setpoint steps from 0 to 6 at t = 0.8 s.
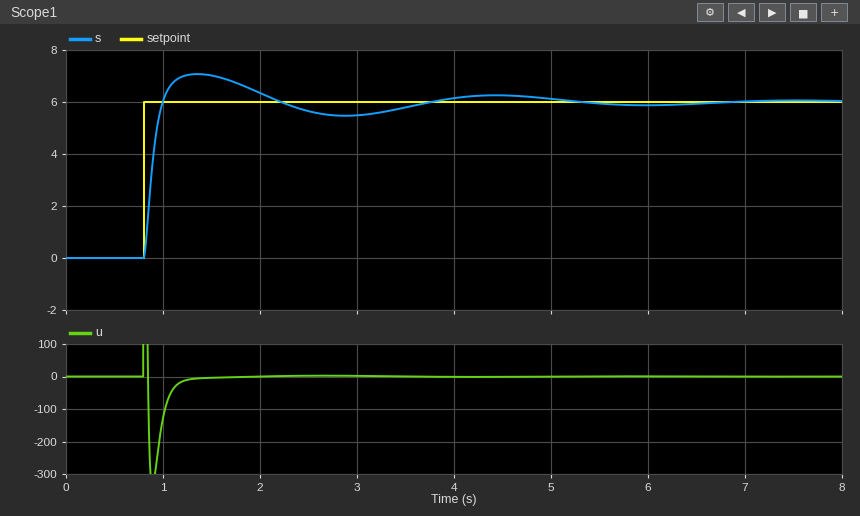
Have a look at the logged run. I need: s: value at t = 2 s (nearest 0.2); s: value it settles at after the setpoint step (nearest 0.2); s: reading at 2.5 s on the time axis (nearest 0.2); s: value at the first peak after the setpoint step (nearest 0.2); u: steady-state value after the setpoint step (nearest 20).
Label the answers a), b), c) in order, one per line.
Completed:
a) 6.4
b) 6.0
c) 5.6
d) 7.0
e) 0
